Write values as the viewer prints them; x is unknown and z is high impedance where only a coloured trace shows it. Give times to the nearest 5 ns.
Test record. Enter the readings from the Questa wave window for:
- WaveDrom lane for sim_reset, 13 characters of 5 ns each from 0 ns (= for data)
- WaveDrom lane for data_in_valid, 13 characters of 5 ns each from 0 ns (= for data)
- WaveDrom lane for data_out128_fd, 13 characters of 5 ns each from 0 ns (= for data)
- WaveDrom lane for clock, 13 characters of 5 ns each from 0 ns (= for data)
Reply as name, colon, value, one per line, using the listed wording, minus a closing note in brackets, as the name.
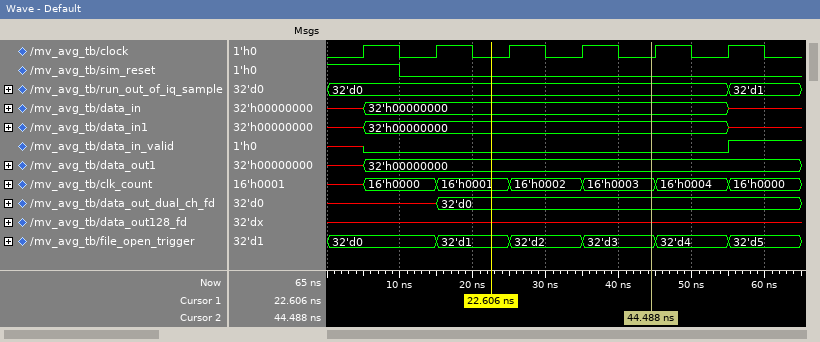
WaveDrom lane for sim_reset, 13 characters of 5 ns each from 0 ns: {name: 'sim_reset', wave: '1.0..........'}
WaveDrom lane for data_in_valid, 13 characters of 5 ns each from 0 ns: {name: 'data_in_valid', wave: 'x0.........1.'}
WaveDrom lane for data_out128_fd, 13 characters of 5 ns each from 0 ns: {name: 'data_out128_fd', wave: 'x............'}
WaveDrom lane for clock, 13 characters of 5 ns each from 0 ns: {name: 'clock', wave: '0101010101010'}
